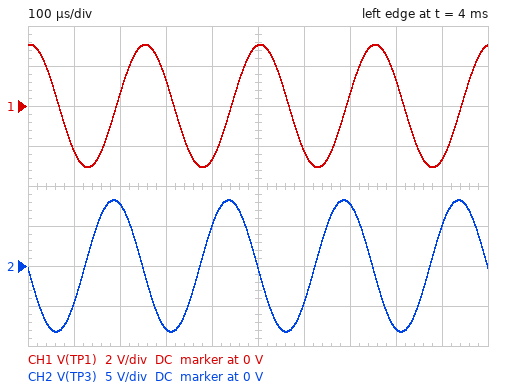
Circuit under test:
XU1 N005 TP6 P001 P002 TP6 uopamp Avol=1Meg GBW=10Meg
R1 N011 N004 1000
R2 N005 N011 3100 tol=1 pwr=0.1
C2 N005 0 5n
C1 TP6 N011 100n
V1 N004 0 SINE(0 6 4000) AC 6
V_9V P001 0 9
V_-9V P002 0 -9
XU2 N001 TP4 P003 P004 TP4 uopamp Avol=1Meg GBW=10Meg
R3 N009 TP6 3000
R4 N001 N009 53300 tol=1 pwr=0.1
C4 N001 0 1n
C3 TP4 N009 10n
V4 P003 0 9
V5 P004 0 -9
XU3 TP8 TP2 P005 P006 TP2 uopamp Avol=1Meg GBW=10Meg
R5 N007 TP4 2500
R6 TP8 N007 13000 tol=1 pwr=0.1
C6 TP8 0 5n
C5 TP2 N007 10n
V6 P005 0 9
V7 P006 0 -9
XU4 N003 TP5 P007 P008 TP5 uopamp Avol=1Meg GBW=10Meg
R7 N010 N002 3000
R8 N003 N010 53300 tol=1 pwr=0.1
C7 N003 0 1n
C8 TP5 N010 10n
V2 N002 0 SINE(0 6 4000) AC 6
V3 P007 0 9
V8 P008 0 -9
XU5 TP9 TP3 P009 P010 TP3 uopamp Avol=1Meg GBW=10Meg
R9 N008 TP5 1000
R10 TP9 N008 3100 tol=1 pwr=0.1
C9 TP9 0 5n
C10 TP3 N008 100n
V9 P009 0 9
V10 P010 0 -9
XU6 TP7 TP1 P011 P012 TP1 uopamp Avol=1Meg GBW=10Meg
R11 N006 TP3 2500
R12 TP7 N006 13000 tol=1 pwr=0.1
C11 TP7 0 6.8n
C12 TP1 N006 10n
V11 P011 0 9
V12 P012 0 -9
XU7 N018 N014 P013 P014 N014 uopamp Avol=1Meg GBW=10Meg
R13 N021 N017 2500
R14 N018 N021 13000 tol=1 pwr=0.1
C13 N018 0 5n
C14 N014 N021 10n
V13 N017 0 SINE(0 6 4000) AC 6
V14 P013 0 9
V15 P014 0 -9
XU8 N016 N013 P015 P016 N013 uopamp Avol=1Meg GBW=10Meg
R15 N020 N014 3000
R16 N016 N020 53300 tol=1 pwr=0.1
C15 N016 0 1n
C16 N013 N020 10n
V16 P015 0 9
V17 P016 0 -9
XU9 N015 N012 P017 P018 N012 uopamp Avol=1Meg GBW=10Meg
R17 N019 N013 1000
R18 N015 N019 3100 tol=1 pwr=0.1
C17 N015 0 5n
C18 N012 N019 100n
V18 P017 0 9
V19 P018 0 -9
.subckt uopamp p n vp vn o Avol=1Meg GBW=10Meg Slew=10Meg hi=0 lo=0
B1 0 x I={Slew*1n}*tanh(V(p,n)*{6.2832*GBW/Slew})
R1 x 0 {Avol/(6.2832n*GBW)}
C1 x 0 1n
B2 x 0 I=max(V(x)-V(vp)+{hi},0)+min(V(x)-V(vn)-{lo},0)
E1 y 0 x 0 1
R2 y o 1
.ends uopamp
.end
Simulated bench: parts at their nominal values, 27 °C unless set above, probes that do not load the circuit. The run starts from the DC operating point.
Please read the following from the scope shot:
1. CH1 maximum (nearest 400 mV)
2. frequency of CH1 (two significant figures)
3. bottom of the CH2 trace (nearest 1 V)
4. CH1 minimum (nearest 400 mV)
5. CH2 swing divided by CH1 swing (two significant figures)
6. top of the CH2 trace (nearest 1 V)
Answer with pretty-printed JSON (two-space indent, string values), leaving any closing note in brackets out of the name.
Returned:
{
  "CH1 maximum": "3.2 V",
  "frequency of CH1": "4.0 kHz",
  "bottom of the CH2 trace": "-8 V",
  "CH1 minimum": "-3.2 V",
  "CH2 swing divided by CH1 swing": "2.7",
  "top of the CH2 trace": "8 V"
}
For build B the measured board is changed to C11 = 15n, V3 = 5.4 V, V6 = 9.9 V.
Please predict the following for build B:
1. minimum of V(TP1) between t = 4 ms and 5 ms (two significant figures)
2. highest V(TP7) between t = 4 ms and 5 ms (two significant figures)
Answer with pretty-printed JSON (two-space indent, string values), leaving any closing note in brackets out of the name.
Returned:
{
  "minimum of V(TP1) between t = 4 ms and 5 ms": "-1.3 V",
  "highest V(TP7) between t = 4 ms and 5 ms": "1.3 V"
}
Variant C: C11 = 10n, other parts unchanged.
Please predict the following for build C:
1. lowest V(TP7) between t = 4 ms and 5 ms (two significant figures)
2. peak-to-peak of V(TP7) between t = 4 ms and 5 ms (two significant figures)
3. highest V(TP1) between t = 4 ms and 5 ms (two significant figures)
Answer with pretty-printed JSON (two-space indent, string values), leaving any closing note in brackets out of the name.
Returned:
{
  "lowest V(TP7) between t = 4 ms and 5 ms": "-2.0 V",
  "peak-to-peak of V(TP7) between t = 4 ms and 5 ms": "4.1 V",
  "highest V(TP1) between t = 4 ms and 5 ms": "2.0 V"
}
